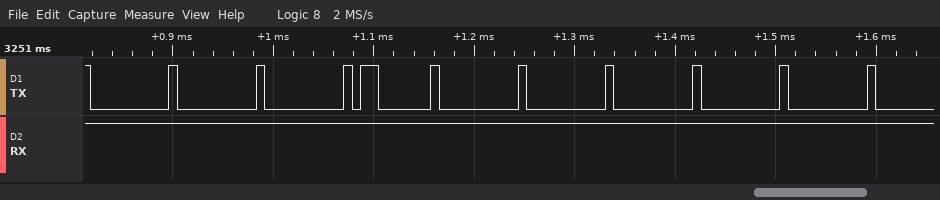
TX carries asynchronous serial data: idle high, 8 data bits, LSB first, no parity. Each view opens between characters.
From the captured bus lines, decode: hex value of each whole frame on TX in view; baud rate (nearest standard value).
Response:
00, 00, 00, 03, 00, 00, 00, 00, 00
115200 baud
